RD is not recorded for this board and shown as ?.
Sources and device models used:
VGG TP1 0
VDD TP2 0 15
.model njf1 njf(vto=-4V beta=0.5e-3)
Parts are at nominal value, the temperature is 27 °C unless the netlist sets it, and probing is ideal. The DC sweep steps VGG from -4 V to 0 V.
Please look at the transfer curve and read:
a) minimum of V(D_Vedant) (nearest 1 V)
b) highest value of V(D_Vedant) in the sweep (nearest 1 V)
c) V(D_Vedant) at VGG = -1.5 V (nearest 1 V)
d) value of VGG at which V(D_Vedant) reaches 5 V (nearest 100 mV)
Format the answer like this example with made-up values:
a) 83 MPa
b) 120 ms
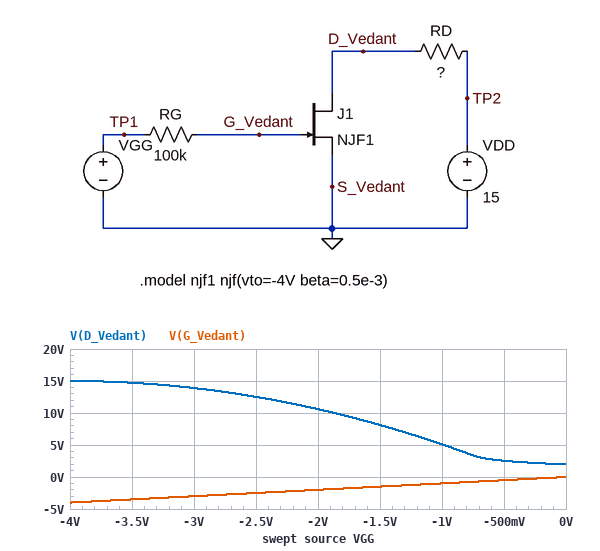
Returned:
a) 2 V
b) 15 V
c) 8 V
d) -1.0 V
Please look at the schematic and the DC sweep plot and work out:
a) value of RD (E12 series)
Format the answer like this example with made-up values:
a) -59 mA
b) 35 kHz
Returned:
a) 2.2 kΩ
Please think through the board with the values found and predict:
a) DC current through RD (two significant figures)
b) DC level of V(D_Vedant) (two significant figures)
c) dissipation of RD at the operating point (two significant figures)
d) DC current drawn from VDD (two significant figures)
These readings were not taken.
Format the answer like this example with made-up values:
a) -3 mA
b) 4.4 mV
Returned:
a) 5.9 mA
b) 2.0 V
c) 77 mW
d) 5.9 mA
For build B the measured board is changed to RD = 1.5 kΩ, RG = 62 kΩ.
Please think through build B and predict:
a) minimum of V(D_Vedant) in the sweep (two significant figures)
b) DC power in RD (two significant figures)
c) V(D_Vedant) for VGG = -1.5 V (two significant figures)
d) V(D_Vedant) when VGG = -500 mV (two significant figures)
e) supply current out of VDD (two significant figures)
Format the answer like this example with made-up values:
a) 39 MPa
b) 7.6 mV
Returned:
a) 3.3 V
b) 91 mW
c) 10 V
d) 5.8 V
e) 7.8 mA
